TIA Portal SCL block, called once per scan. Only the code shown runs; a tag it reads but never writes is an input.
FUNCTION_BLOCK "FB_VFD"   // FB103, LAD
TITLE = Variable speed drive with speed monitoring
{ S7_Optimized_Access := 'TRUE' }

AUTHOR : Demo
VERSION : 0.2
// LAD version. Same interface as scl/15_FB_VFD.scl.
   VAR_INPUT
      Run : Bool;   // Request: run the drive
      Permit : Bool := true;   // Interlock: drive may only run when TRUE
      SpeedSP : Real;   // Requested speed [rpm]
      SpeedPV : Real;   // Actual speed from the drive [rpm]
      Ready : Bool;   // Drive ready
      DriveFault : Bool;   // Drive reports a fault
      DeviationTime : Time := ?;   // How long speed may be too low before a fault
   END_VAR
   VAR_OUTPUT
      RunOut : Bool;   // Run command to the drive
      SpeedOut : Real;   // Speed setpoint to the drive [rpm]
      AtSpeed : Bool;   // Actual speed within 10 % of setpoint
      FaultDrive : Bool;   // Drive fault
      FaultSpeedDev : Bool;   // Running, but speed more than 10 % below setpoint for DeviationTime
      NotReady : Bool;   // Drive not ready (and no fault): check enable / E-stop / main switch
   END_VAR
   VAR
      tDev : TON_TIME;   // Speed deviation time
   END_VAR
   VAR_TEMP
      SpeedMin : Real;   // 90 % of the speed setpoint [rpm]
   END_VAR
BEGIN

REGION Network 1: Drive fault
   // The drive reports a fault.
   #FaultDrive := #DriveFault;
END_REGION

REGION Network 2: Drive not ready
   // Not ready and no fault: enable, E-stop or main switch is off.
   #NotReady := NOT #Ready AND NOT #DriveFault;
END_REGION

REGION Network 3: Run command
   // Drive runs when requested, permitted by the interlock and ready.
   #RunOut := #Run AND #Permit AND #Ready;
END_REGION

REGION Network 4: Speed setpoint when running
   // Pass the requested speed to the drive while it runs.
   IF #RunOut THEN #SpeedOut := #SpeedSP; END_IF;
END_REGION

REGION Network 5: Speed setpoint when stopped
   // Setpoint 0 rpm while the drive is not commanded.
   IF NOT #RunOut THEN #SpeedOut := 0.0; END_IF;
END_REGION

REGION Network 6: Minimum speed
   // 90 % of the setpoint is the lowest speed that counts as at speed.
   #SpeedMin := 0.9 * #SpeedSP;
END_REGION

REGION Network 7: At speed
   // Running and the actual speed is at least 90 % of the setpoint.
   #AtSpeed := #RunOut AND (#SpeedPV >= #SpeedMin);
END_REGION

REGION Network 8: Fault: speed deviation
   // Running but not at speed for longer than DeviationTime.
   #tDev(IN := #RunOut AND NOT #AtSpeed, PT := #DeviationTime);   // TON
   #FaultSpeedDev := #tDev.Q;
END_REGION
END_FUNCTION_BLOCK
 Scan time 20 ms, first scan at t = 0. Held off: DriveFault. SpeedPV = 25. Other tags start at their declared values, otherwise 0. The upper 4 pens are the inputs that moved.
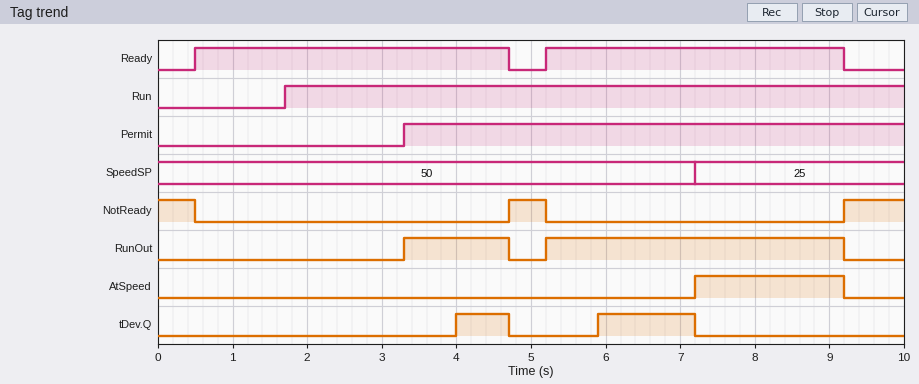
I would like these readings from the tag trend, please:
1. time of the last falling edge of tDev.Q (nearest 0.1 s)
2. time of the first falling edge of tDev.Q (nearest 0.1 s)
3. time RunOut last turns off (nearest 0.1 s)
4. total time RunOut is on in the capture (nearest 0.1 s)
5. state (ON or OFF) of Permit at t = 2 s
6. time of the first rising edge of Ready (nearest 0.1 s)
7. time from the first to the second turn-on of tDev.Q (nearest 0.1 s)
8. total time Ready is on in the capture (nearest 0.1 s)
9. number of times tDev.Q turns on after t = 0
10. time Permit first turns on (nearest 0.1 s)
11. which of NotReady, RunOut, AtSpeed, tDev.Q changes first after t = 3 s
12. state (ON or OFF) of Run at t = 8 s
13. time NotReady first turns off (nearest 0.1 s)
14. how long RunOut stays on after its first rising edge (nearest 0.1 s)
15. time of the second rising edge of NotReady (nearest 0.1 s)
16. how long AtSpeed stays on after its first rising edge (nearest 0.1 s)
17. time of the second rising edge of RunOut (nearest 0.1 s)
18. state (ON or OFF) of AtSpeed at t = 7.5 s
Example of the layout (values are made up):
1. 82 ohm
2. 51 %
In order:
1. 7.2 s
2. 4.7 s
3. 9.2 s
4. 5.4 s
5. OFF
6. 0.5 s
7. 1.9 s
8. 8.2 s
9. 2
10. 3.3 s
11. RunOut
12. ON
13. 0.5 s
14. 1.4 s
15. 9.2 s
16. 2.0 s
17. 5.2 s
18. ON
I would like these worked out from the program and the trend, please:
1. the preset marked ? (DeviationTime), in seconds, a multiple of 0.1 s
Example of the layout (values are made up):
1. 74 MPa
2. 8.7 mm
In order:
1. 0.7 s
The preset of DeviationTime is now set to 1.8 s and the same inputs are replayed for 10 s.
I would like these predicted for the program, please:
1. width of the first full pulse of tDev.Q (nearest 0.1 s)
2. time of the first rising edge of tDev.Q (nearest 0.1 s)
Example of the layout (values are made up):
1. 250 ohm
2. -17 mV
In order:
1. 0.2 s
2. 7.0 s
